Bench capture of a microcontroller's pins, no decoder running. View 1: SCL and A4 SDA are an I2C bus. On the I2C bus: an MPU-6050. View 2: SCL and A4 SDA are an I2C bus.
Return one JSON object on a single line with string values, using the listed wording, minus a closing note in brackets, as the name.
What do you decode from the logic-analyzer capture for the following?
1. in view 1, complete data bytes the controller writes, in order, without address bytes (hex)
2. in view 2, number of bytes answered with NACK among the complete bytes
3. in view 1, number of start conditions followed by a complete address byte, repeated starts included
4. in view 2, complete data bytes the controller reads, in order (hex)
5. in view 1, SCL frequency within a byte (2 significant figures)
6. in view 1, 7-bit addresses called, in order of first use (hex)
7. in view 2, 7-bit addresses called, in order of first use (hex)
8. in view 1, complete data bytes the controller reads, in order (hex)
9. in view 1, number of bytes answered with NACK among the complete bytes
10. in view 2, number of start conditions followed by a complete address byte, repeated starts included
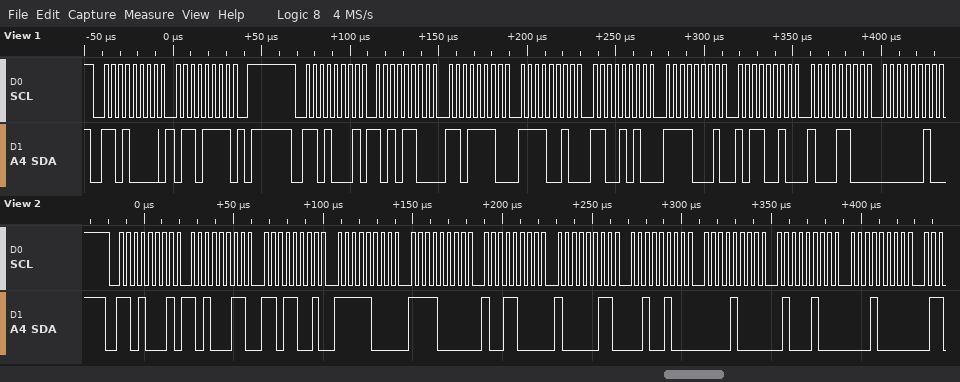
{"in view 1, complete data bytes the controller writes, in order, without address bytes": "6F", "in view 2, number of bytes answered with NACK among the complete bytes": "0", "in view 1, number of start conditions followed by a complete address byte, repeated starts included": "2", "in view 2, complete data bytes the controller reads, in order": "A3 D9 F8 F0 98 83 24 08 44 10", "in view 1, SCL frequency within a byte": "250 kHz", "in view 1, 7-bit addresses called, in order of first use": "0x68", "in view 2, 7-bit addresses called, in order of first use": "0x68", "in view 1, complete data bytes the controller reads, in order": "AC DE F2 CA F1 B2 8C 02", "in view 1, number of bytes answered with NACK among the complete bytes": "0", "in view 2, number of start conditions followed by a complete address byte, repeated starts included": "1"}
